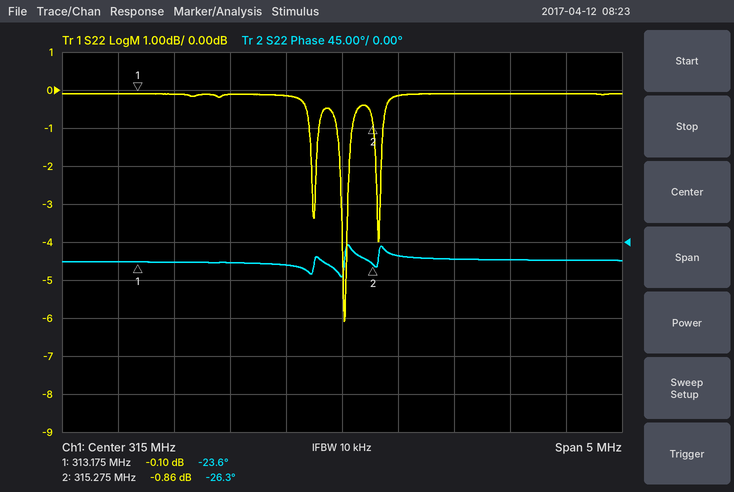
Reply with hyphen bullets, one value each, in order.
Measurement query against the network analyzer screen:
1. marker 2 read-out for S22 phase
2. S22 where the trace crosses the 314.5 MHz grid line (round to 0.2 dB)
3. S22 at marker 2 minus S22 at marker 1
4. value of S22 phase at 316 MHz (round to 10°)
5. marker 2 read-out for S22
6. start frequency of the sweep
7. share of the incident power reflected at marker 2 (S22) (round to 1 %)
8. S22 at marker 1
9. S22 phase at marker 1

- -26.3°
- -0.2 dB
- -0.76 dB
- -20°
- -0.86 dB
- 312.5 MHz
- 82 %
- -0.10 dB
- -23.6°
